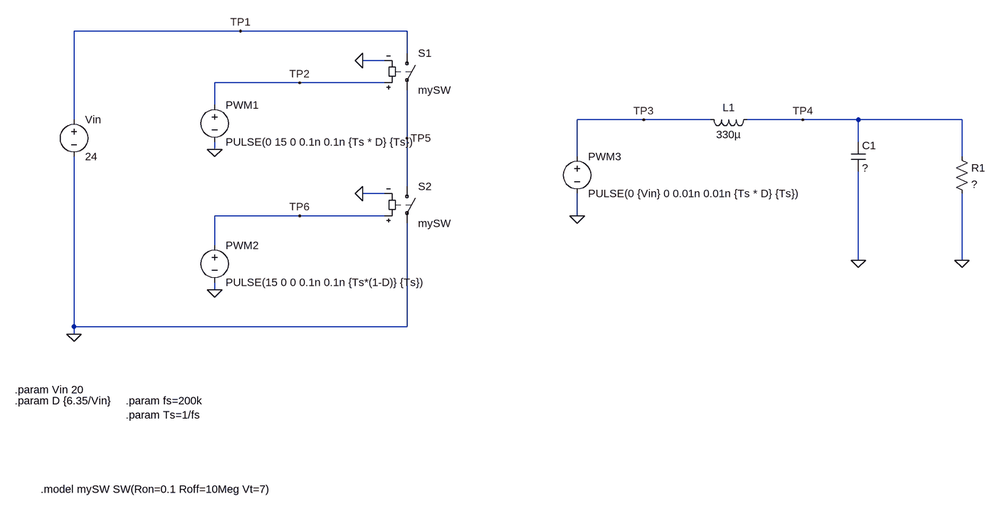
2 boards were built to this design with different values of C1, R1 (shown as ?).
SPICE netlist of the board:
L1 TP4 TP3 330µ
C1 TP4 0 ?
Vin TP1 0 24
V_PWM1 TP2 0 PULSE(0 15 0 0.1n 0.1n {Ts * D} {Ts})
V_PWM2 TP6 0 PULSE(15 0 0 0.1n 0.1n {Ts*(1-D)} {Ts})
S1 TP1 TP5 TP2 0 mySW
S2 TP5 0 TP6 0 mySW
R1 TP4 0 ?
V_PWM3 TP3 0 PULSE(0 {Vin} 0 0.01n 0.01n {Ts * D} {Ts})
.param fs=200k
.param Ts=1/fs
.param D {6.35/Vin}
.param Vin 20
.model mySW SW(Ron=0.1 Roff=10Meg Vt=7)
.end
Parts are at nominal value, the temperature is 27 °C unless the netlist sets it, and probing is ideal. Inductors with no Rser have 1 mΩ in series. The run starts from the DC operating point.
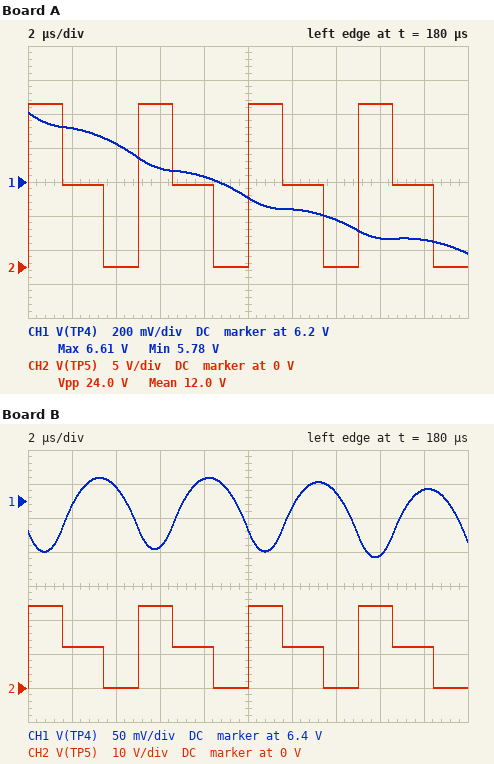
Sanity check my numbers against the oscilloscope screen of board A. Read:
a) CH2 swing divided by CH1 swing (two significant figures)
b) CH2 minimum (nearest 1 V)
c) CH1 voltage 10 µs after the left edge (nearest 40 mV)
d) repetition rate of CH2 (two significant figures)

29
0 V
6.12 V
200 kHz
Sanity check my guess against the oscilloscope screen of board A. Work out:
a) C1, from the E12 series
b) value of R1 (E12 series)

820 nF
56 Ω
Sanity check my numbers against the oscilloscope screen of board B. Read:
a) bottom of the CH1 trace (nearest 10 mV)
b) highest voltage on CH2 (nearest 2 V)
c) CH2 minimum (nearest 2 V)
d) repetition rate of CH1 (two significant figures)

6.32 V
24 V
0 V
200 kHz
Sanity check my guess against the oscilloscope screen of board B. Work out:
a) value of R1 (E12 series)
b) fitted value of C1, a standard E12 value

47 Ω
390 nF
